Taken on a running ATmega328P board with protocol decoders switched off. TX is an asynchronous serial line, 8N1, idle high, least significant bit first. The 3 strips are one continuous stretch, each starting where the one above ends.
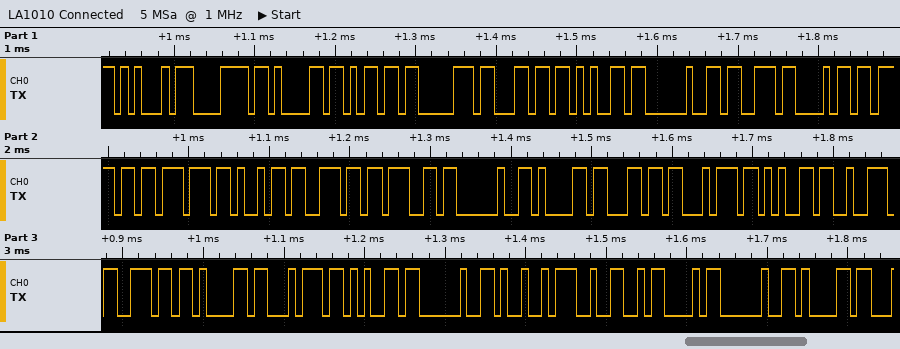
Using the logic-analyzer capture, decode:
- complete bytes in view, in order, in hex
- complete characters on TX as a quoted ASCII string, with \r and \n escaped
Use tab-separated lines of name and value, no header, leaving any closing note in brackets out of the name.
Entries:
complete bytes in view, in order, in hex	45 78 61 6D 70 6C 65 20 73 68 6F 77 69 6E 67 20 61 6C 74 65 72 6E 61 74 65 20 49 32 43 20 61
complete characters on TX as a quoted ASCII string, with \r and \n escaped	"Example showing alternate I2C a"
